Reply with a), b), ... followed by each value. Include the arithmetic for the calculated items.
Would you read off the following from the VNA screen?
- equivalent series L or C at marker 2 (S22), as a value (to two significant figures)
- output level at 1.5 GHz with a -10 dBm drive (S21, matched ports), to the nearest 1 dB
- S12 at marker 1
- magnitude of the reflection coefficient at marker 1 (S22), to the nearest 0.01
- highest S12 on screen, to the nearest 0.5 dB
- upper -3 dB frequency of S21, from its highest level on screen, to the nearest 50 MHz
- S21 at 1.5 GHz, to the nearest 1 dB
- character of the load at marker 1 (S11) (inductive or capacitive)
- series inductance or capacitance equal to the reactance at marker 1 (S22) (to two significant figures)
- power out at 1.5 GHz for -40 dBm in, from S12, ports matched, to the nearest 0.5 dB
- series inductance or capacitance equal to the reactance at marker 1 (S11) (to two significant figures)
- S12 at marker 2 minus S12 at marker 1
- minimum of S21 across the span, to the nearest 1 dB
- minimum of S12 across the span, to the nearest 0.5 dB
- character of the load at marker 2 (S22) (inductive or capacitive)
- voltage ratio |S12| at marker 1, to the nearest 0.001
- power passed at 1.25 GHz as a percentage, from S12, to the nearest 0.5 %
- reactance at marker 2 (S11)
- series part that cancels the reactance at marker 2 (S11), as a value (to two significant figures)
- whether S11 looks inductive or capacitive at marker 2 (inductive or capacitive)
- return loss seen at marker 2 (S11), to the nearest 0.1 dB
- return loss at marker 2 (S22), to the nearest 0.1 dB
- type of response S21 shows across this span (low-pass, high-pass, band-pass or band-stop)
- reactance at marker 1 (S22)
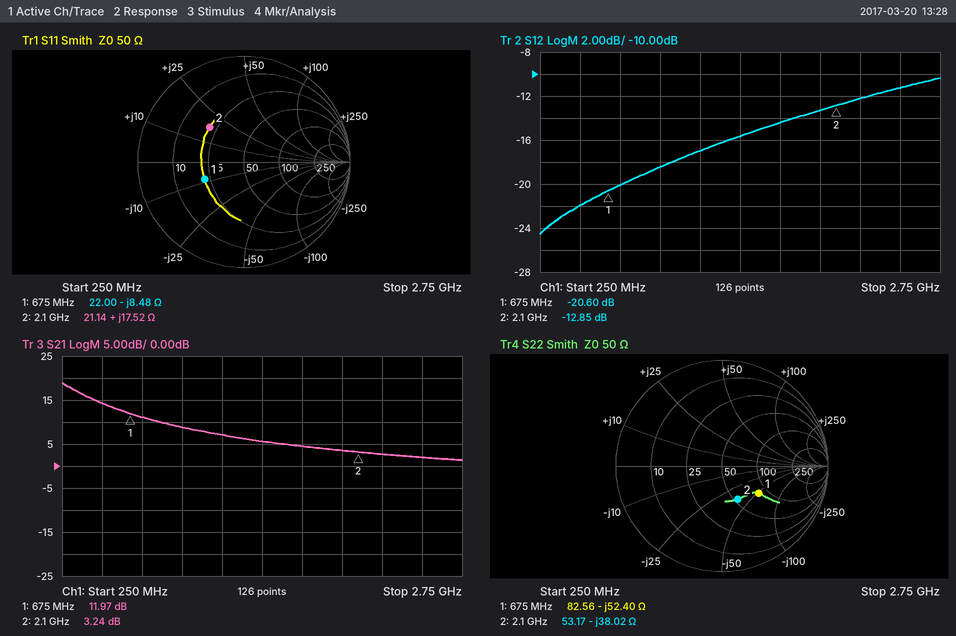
a) C = 1/(2π × 2.1 GHz × 38.02 Ω) ≈ 2.0 pF
b) -10 dBm + (6 dB) = -4 dBm
c) -20.60 dB
d) 0.43
e) -10.5 dB
f) 400 MHz
g) 6 dB
h) capacitive
i) C = 1/(2π × 675 MHz × 52.4 Ω) ≈ 4.5 pF
j) -40 dBm + (-15.5 dB) = -55.5 dBm
k) C = 1/(2π × 675 MHz × 8.48 Ω) ≈ 28 pF
l) -12.85 − (-20.6) = 7.75 dB
m) 1 dB
n) -24.5 dB
o) capacitive
p) 10^(-20.6/20) ≈ 0.093
q) 10^(-17/10) ≈ 2.0 %
r) +17.52 Ω
s) C = 1/(2π × 2.1 GHz × 17.52 Ω) ≈ 4.3 pF
t) inductive
u) 6.7 dB
v) 9.2 dB
w) low-pass
x) -52.40 Ω
